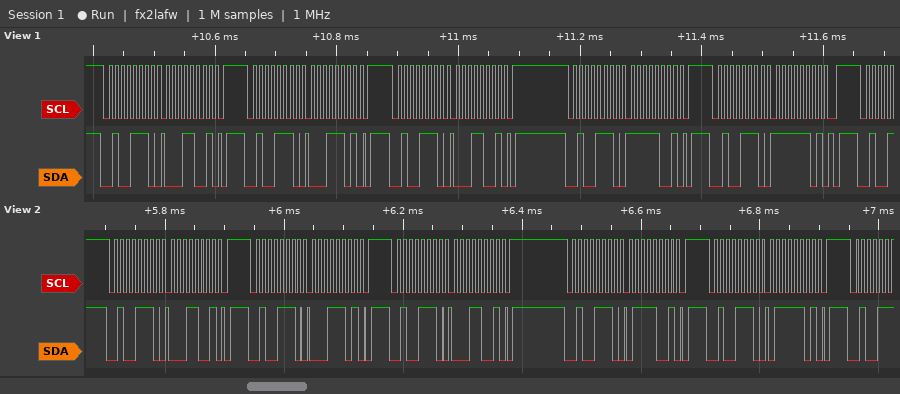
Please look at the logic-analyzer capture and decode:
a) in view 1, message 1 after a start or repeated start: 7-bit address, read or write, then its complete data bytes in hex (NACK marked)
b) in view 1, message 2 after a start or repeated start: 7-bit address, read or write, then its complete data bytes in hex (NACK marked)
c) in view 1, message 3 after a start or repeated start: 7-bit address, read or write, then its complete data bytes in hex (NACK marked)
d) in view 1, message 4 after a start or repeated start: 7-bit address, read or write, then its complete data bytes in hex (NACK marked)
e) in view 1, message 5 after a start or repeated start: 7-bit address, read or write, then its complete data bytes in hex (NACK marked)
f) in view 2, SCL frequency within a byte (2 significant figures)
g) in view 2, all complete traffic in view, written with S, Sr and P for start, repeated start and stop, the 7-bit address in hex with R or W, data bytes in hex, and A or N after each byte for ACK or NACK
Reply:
0x27 write: 19
0x27 write: 1D
0x27 write: 19
0x27 write: F9
0x27 write: FD
100 kHz
S 27W A 19 A P S 27W A 1D A P S 27W A 19 A P S 27W A 79 A P S 27W A 7D A P
